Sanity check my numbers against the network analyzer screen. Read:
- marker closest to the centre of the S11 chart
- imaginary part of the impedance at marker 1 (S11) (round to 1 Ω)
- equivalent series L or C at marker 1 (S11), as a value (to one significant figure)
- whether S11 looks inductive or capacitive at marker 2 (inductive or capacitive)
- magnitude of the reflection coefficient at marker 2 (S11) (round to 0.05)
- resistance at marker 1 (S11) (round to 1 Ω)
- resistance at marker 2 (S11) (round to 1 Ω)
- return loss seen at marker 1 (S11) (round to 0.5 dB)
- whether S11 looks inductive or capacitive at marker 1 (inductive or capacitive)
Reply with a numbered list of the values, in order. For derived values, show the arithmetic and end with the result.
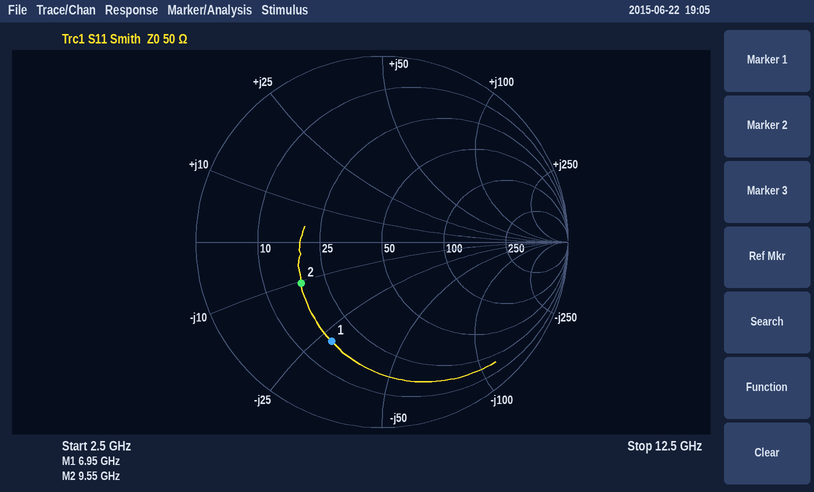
1. marker 2
2. -28 Ω
3. C = 1/(2π × 6.95 GHz × 28 Ω) ≈ 818 fF, so 800 fF to one significant figure
4. capacitive
5. 0.50
6. 17 Ω
7. 18 Ω
8. 4.5 dB
9. capacitive
